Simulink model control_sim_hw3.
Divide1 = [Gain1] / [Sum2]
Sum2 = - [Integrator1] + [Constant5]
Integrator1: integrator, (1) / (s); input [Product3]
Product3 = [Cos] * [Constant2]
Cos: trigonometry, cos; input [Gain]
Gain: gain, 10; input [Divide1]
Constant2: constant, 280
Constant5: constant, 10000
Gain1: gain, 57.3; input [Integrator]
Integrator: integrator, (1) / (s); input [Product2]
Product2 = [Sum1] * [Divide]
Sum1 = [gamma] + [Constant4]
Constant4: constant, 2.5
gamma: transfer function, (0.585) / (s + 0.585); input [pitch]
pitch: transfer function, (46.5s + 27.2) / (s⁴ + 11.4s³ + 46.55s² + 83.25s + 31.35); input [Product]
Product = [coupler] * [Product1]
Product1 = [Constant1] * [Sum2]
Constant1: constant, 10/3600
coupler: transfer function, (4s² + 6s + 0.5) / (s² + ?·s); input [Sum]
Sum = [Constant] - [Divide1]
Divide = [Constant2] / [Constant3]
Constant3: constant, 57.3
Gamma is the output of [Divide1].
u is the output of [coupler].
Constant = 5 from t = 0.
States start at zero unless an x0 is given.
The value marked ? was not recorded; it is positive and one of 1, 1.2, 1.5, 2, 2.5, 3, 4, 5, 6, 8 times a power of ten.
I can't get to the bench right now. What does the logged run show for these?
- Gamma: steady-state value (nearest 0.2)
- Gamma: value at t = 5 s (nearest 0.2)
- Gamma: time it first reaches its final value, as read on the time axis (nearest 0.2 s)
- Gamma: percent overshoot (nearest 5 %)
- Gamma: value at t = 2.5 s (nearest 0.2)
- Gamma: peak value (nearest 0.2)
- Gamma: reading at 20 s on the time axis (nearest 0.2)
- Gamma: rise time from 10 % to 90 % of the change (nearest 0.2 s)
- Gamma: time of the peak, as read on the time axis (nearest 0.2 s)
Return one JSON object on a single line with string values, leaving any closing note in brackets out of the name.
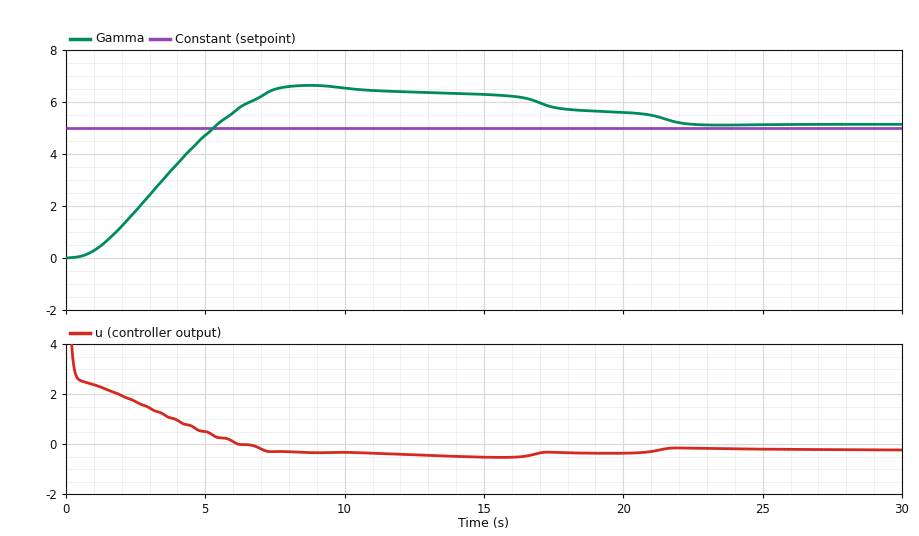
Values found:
{"Gamma: steady-state value": "5.2", "Gamma: value at t = 5 s": "4.8", "Gamma: time it first reaches its final value, as read on the time axis": "5.4 s", "Gamma: percent overshoot": "30 %", "Gamma: value at t = 2.5 s": "1.8", "Gamma: peak value": "6.6", "Gamma: reading at 20 s on the time axis": "5.6", "Gamma: rise time from 10 % to 90 % of the change": "3.6 s", "Gamma: time of the peak, as read on the time axis": "8.8 s"}
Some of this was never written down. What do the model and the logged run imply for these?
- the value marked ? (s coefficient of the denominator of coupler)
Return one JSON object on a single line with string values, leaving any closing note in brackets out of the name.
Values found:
{"the value marked ?": "12"}
